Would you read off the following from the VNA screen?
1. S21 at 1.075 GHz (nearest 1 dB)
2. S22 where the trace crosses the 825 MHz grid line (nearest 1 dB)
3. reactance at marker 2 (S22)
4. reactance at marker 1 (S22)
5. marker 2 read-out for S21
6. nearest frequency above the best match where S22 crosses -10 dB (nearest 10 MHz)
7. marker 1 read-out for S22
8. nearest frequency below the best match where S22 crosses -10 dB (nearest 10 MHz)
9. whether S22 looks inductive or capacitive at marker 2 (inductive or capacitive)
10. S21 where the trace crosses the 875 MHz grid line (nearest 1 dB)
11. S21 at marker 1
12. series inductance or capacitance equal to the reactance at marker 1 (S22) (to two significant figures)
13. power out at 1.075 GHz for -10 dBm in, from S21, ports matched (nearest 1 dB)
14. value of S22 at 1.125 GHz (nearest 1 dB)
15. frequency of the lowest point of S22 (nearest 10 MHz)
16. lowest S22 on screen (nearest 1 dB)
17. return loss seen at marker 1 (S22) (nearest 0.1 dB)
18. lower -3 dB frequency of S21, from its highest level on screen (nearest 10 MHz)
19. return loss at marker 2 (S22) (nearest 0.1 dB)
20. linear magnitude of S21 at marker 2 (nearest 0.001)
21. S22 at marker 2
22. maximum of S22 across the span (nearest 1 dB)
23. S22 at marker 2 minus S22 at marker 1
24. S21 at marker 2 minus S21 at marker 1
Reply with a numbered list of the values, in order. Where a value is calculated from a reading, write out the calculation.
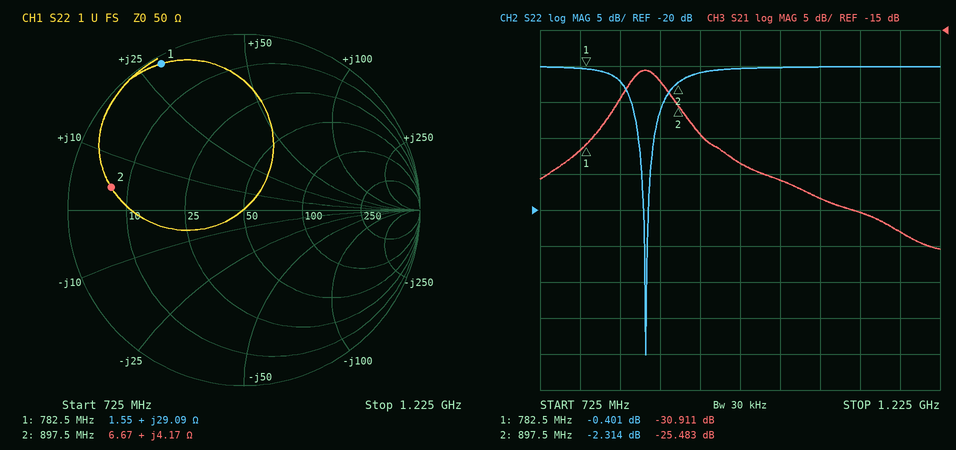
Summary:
1. -38 dB
2. -2 dB
3. +4.17 Ω
4. +29.09 Ω
5. -25.483 dB
6. 870 MHz
7. -0.401 dB
8. 850 MHz
9. inductive
10. -22 dB
11. -30.911 dB
12. L = 29.09 Ω/(2π × 782.5 MHz) ≈ 5.9 nH
13. -10 dBm + (-38 dB) = -48 dBm
14. 0 dB
15. 860 MHz
16. -40 dB
17. 0.4 dB
18. 830 MHz
19. 2.3 dB
20. 10^(-25.483/20) ≈ 0.053
21. -2.314 dB
22. 0 dB
23. -2.314 − (-0.401) = -1.913 dB
24. -25.483 − (-30.911) = 5.428 dB
